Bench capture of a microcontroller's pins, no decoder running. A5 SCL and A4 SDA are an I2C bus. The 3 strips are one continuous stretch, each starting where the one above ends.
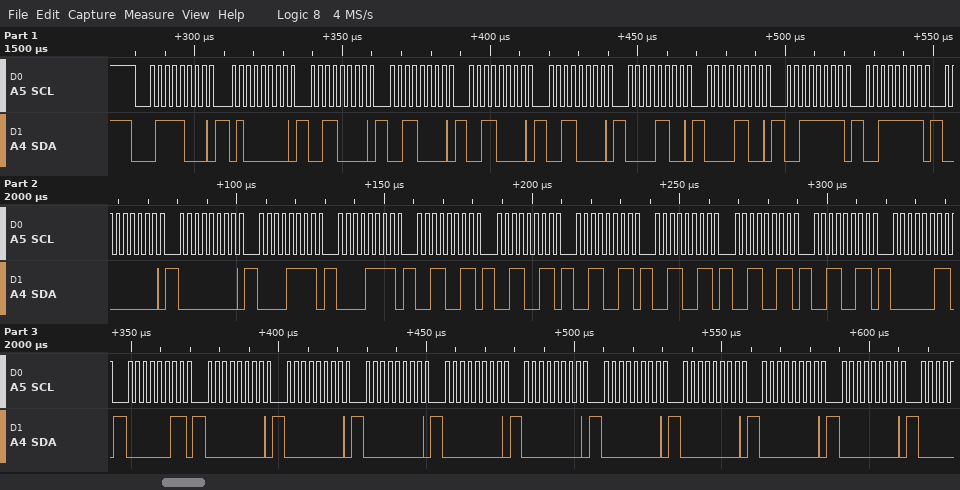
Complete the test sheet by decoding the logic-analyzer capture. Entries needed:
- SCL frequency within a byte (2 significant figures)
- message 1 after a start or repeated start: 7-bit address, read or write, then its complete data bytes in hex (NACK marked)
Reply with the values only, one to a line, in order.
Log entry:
400 kHz
0x3C write: 40 30 30 30 30 0C 0C 3F 3F 00 00 0F 0F 33 33 33 33 33 33 03 03 00 00 00 00 00 00 00 00 00
